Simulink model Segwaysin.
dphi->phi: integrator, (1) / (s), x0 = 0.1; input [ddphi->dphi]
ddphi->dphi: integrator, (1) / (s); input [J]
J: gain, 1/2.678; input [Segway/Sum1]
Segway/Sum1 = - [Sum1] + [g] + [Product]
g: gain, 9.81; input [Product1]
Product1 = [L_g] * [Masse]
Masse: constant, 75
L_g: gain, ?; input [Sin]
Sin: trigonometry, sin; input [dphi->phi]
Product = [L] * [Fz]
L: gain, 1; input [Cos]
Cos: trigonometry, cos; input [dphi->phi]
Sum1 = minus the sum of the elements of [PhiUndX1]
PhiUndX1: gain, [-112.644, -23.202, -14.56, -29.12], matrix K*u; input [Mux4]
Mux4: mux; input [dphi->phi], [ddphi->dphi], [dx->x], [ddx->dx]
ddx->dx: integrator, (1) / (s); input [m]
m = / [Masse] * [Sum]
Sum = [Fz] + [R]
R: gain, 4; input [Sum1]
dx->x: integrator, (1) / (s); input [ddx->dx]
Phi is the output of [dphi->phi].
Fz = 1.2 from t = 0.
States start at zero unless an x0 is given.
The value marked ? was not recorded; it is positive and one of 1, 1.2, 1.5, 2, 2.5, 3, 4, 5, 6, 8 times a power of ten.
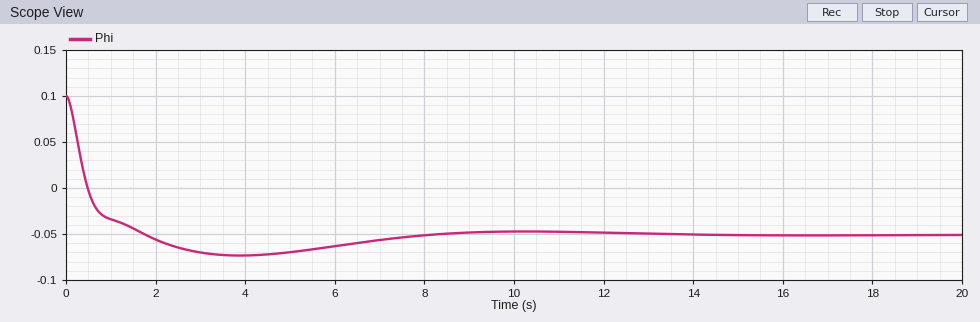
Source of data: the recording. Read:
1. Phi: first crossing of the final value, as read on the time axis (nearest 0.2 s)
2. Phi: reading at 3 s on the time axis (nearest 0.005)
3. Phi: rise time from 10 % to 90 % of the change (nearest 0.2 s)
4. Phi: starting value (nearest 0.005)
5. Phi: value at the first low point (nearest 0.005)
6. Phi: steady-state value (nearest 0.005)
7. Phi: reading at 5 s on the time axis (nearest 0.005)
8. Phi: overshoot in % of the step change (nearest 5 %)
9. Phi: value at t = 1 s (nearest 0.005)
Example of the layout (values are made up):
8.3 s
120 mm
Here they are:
1.8 s
-0.070
1.0 s
0.100
-0.075
-0.050
-0.070
15 %
-0.035
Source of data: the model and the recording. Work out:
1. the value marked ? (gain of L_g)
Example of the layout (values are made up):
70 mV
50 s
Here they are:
0.04
